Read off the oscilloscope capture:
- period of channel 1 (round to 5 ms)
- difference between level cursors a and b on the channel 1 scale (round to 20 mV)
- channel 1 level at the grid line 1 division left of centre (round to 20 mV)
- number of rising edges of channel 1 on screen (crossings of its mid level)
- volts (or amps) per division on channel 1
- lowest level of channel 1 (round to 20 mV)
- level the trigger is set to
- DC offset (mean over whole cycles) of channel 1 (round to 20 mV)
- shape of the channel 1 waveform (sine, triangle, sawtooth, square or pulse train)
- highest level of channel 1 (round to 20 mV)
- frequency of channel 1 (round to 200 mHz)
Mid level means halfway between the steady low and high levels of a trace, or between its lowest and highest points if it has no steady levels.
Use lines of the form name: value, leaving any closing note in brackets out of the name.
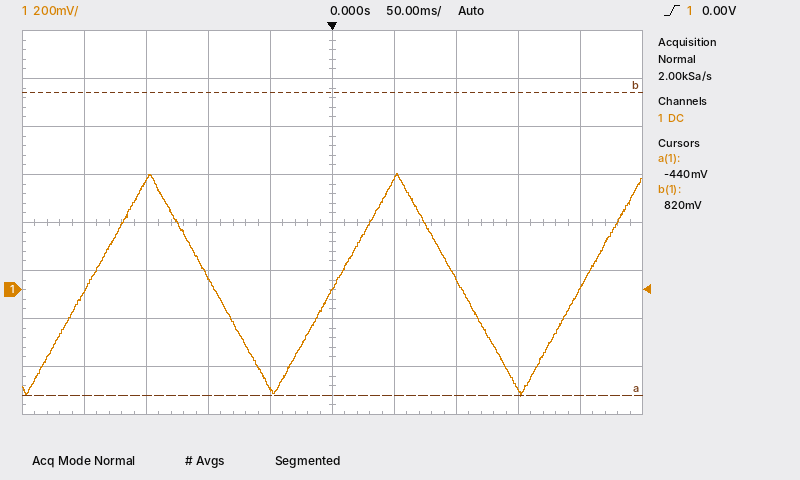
period of channel 1: 200 ms
difference between level cursors a and b on the channel 1 scale: 1.26 V
channel 1 level at the grid line 1 division left of centre: -420 mV
number of rising edges of channel 1 on screen: 3
volts (or amps) per division on channel 1: 200 mV
lowest level of channel 1: -440 mV
level the trigger is set to: 0.00 V
DC offset (mean over whole cycles) of channel 1: 20 mV
shape of the channel 1 waveform: triangle
highest level of channel 1: 480 mV
frequency of channel 1: 5.0 Hz
